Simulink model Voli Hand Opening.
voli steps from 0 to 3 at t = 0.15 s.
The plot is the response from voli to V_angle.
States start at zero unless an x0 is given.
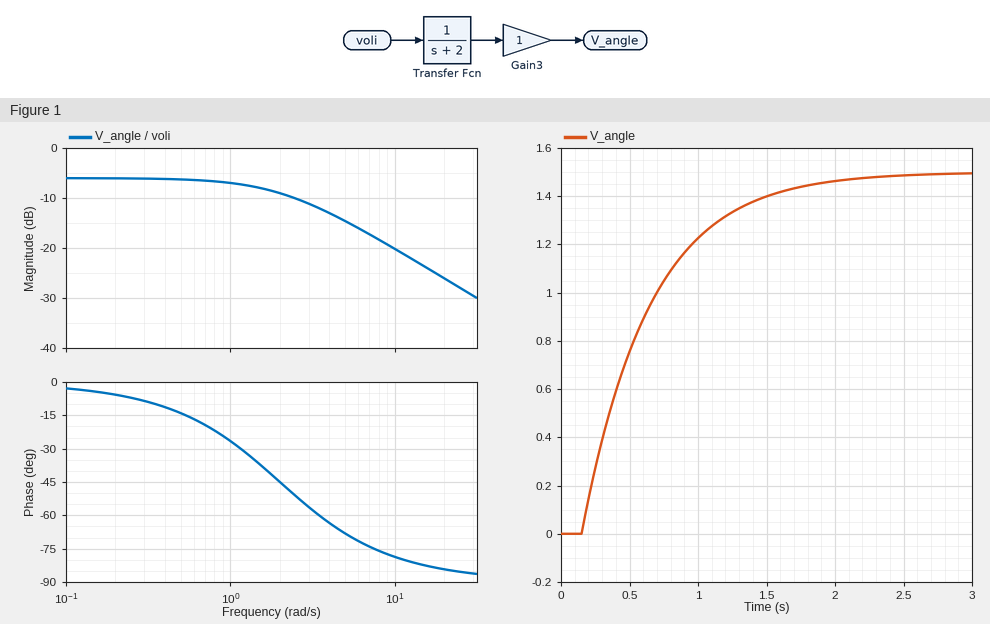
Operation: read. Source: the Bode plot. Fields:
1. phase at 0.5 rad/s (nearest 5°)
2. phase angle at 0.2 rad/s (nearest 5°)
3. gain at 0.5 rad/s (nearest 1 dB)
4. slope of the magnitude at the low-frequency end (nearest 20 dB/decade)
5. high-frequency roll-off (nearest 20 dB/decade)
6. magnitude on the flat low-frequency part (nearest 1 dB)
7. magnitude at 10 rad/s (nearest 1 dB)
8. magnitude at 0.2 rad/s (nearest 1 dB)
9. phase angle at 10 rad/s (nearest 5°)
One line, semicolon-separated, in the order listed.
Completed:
-15°; -5°; -6 dB; 0 dB/decade; -20 dB/decade; -6 dB; -20 dB; -6 dB; -80°
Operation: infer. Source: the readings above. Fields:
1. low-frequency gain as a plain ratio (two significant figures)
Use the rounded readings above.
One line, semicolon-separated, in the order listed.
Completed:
0.50
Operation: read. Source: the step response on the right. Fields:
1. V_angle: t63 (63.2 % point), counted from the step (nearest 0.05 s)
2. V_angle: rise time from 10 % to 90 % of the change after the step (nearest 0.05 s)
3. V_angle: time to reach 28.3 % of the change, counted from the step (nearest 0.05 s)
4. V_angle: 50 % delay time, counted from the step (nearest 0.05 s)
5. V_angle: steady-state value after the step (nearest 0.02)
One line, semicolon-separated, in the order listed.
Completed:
0.50 s; 1.10 s; 0.15 s; 0.35 s; 1.50
